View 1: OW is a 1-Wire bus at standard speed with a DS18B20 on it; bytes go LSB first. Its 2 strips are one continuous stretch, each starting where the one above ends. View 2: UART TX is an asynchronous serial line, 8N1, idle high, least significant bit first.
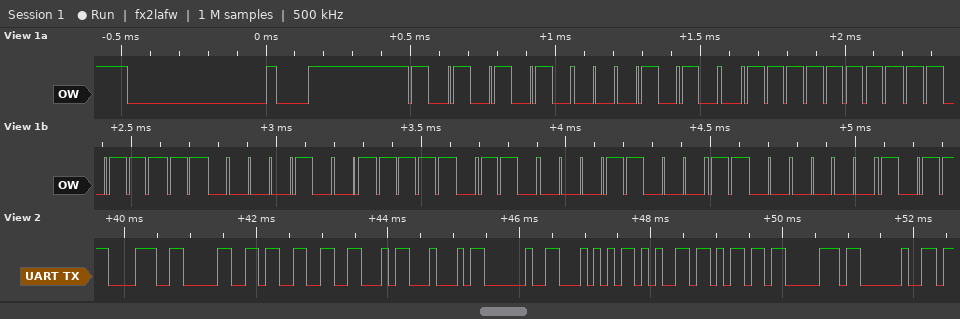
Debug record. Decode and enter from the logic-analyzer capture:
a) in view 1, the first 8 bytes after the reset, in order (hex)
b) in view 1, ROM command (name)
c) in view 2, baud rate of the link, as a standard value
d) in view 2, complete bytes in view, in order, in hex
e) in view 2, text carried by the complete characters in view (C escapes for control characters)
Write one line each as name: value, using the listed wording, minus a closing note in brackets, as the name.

in view 1, the first 8 bytes after the reset, in order: 55 28 FF FB 90 6F 18 03
in view 1, ROM command: Match ROM
in view 2, baud rate of the link, as a standard value: 9600 baud
in view 2, complete bytes in view, in order, in hex: 0x38 0x30 0x33 0x46 0x44 0x20 0x54 0x65 0x6D 0x70 0x20
in view 2, text carried by the complete characters in view: "803FD Temp "
